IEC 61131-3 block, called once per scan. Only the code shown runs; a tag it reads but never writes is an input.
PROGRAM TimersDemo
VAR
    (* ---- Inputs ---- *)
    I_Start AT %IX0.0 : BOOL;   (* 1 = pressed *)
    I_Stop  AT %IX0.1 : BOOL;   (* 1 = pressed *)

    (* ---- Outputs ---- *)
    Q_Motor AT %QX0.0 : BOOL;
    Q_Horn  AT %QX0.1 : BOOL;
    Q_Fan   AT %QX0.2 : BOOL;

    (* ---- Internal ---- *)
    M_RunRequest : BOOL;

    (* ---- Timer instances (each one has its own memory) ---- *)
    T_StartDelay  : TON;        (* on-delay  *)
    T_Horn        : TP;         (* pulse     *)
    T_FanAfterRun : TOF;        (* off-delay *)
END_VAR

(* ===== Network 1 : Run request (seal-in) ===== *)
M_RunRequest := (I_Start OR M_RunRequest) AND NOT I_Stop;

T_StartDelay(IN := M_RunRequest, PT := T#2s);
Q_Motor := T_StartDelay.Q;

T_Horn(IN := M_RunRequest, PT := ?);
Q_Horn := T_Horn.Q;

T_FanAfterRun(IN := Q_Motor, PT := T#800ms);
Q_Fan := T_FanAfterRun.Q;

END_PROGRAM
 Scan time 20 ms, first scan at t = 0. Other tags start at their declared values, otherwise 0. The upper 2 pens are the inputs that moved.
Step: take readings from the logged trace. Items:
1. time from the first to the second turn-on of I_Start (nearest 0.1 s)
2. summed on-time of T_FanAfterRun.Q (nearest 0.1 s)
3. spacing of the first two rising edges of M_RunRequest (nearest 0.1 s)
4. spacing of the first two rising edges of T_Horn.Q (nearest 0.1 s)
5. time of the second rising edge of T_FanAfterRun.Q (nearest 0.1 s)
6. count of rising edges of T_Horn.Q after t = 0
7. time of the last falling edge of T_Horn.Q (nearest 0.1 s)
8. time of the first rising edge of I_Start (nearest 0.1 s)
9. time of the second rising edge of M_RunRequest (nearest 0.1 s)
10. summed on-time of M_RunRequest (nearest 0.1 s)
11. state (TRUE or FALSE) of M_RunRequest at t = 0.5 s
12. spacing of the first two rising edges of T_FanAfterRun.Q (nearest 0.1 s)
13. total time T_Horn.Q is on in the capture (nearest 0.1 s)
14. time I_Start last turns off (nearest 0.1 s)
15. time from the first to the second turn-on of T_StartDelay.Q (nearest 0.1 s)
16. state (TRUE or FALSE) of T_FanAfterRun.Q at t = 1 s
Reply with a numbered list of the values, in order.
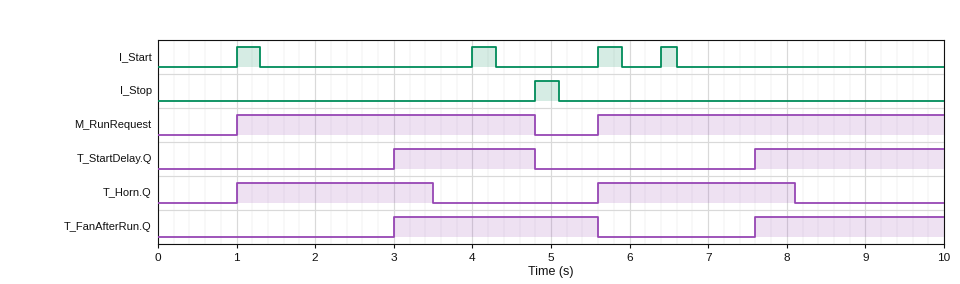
1. 3.0 s
2. 5.0 s
3. 4.6 s
4. 4.6 s
5. 7.6 s
6. 2
7. 8.1 s
8. 1.0 s
9. 5.6 s
10. 8.2 s
11. FALSE
12. 4.6 s
13. 5.0 s
14. 6.6 s
15. 4.6 s
16. FALSE
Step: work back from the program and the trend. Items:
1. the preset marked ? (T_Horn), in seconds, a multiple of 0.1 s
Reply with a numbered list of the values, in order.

1. 2.5 s
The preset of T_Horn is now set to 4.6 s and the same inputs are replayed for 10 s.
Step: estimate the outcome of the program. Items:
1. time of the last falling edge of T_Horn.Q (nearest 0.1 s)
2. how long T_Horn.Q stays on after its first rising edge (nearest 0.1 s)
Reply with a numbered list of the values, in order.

1. 5.6 s
2. 4.6 s
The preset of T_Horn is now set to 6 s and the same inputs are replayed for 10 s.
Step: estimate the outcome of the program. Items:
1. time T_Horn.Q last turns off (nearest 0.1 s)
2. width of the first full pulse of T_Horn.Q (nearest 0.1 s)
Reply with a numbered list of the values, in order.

1. 7.0 s
2. 6.0 s
